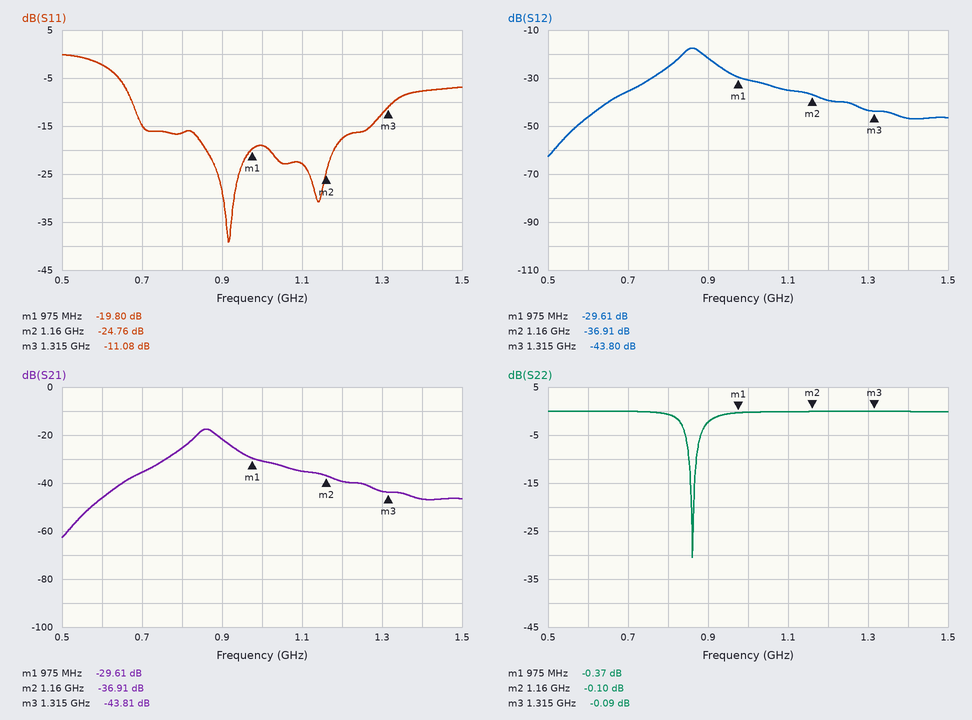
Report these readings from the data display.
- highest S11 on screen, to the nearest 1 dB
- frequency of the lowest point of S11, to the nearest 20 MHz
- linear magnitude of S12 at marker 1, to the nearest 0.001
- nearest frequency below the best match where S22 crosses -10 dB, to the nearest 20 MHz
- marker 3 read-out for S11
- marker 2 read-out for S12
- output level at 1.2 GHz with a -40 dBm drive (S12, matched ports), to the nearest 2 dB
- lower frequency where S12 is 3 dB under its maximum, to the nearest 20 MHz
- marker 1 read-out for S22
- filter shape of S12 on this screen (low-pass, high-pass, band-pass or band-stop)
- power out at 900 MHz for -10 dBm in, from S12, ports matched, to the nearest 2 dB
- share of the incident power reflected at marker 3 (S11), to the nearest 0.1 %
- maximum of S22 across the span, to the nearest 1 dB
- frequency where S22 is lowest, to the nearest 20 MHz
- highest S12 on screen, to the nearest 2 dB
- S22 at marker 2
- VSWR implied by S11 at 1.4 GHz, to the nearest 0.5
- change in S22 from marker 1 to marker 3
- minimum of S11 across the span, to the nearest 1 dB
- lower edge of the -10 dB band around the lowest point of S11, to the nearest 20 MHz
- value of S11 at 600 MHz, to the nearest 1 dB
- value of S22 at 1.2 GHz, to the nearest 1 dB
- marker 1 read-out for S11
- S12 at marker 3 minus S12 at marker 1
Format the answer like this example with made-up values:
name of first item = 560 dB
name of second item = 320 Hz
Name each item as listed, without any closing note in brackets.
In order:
highest S11 on screen, to the nearest 1 dB = 0 dB
frequency of the lowest point of S11, to the nearest 20 MHz = 920 MHz
linear magnitude of S12 at marker 1, to the nearest 0.001 = 0.033
nearest frequency below the best match where S22 crosses -10 dB, to the nearest 20 MHz = 860 MHz
marker 3 read-out for S11 = -11.08 dB
marker 2 read-out for S12 = -36.91 dB
output level at 1.2 GHz with a -40 dBm drive (S12, matched ports), to the nearest 2 dB = -80 dBm
lower frequency where S12 is 3 dB under its maximum, to the nearest 20 MHz = 840 MHz
marker 1 read-out for S22 = -0.37 dB
filter shape of S12 on this screen = band-pass
power out at 900 MHz for -10 dBm in, from S12, ports matched, to the nearest 2 dB = -32 dBm
share of the incident power reflected at marker 3 (S11), to the nearest 0.1 % = 7.8 %
maximum of S22 across the span, to the nearest 1 dB = 0 dB
frequency where S22 is lowest, to the nearest 20 MHz = 860 MHz
highest S12 on screen, to the nearest 2 dB = -18 dB
S22 at marker 2 = -0.10 dB
VSWR implied by S11 at 1.4 GHz, to the nearest 0.5 = 2.5
change in S22 from marker 1 to marker 3 = 0.28 dB
minimum of S11 across the span, to the nearest 1 dB = -39 dB
lower edge of the -10 dB band around the lowest point of S11, to the nearest 20 MHz = 680 MHz
value of S11 at 600 MHz, to the nearest 1 dB = -2 dB
value of S22 at 1.2 GHz, to the nearest 1 dB = 0 dB
marker 1 read-out for S11 = -19.80 dB
S12 at marker 3 minus S12 at marker 1 = -14.19 dB
